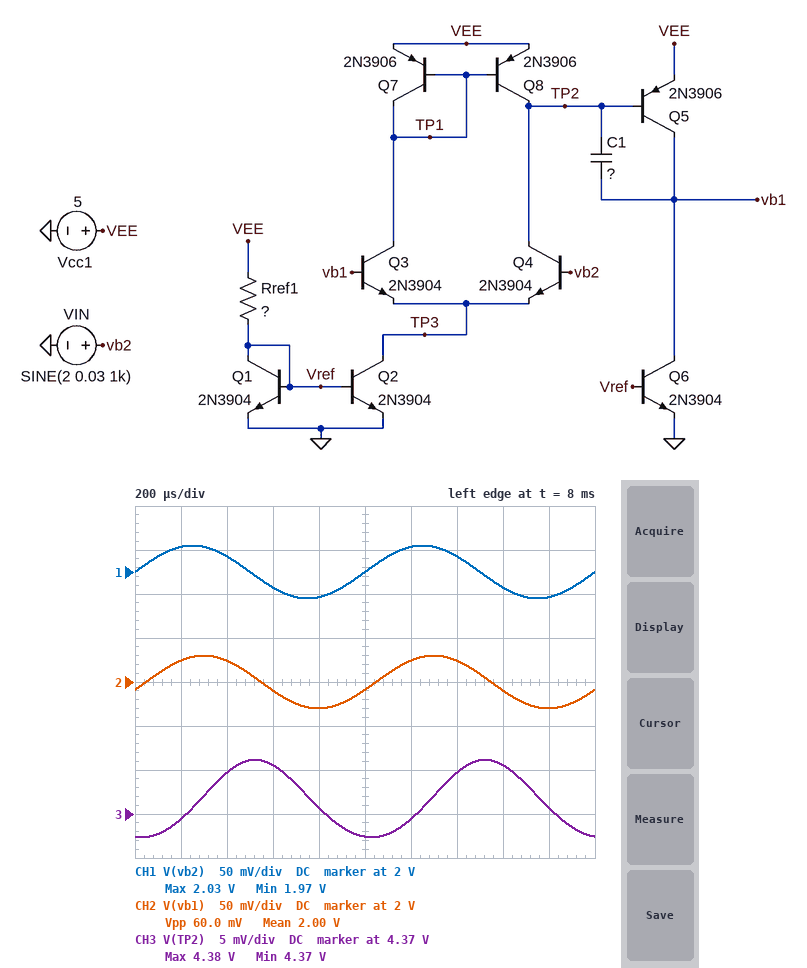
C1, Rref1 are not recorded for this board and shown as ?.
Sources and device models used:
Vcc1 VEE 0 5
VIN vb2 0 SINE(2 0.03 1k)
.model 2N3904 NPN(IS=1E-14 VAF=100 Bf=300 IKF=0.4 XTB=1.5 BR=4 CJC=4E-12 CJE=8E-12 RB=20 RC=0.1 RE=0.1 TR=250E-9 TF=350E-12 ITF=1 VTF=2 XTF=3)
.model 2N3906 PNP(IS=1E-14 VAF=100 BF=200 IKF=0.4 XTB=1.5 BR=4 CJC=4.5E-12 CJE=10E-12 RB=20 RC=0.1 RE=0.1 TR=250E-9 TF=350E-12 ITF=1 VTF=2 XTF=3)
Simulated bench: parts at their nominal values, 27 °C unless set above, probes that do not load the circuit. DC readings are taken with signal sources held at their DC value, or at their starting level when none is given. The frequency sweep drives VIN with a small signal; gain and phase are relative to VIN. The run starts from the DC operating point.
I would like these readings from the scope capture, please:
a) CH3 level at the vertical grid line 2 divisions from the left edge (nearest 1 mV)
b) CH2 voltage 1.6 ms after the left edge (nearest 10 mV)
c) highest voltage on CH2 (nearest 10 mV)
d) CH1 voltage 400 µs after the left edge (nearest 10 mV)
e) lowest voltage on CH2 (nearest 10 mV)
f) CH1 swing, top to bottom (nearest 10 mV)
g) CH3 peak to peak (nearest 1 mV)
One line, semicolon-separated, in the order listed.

4.375 V; 1.99 V; 2.03 V; 2.02 V; 1.97 V; 60 mV; 9 mV
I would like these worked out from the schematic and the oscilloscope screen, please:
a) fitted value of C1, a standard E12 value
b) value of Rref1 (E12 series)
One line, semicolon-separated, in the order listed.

330 nF; 12 kΩ
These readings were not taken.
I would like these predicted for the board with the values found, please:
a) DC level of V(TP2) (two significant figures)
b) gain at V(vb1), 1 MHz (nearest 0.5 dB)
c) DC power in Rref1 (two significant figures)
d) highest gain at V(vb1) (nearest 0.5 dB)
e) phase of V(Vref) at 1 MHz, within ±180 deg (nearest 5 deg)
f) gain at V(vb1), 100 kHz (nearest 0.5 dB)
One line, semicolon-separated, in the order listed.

4.4 V; -0.5 dB; 1.6 mW; 0 dB; -100 deg; -0.5 dB
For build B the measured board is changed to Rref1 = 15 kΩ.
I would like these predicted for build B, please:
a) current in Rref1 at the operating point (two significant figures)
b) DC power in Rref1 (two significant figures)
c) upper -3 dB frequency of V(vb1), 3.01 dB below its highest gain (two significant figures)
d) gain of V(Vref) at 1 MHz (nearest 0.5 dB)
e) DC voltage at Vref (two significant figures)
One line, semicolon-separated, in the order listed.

290 µA; 1.3 mW; 8.8 MHz; -56.5 dB; 620 mV
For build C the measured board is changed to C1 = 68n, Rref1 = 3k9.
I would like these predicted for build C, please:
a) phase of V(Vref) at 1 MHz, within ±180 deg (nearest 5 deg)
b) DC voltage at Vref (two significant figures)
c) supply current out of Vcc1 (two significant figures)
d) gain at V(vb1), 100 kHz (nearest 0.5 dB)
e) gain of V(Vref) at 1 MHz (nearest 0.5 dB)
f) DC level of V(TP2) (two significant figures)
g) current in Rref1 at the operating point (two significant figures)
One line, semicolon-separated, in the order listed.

-75 deg; 660 mV; 3.3 mA; 0 dB; -68.0 dB; 4.3 V; 1.1 mA
